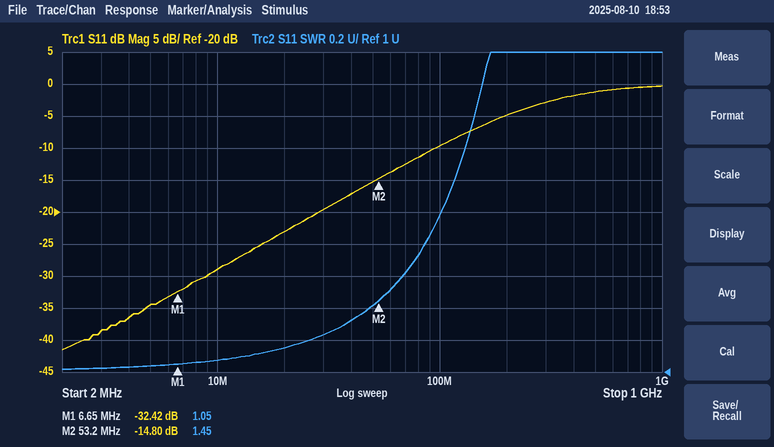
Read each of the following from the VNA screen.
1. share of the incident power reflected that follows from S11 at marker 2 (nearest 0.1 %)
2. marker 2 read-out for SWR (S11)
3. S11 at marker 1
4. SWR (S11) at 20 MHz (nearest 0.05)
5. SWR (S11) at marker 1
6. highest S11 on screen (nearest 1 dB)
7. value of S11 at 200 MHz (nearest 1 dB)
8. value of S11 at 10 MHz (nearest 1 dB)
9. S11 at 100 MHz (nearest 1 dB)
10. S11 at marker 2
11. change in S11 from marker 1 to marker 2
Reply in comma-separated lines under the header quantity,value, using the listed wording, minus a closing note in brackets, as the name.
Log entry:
quantity,value
share of the incident power reflected that follows from S11 at marker 2,3.3 %
marker 2 read-out for SWR,1.45
S11 at marker 1,-32.42 dB
SWR (S11) at 20 MHz,1.15
SWR (S11) at marker 1,1.05
highest S11 on screen,0 dB
value of S11 at 200 MHz,-5 dB
value of S11 at 10 MHz,-29 dB
S11 at 100 MHz,-10 dB
S11 at marker 2,-14.80 dB
change in S11 from marker 1 to marker 2,17.62 dB
